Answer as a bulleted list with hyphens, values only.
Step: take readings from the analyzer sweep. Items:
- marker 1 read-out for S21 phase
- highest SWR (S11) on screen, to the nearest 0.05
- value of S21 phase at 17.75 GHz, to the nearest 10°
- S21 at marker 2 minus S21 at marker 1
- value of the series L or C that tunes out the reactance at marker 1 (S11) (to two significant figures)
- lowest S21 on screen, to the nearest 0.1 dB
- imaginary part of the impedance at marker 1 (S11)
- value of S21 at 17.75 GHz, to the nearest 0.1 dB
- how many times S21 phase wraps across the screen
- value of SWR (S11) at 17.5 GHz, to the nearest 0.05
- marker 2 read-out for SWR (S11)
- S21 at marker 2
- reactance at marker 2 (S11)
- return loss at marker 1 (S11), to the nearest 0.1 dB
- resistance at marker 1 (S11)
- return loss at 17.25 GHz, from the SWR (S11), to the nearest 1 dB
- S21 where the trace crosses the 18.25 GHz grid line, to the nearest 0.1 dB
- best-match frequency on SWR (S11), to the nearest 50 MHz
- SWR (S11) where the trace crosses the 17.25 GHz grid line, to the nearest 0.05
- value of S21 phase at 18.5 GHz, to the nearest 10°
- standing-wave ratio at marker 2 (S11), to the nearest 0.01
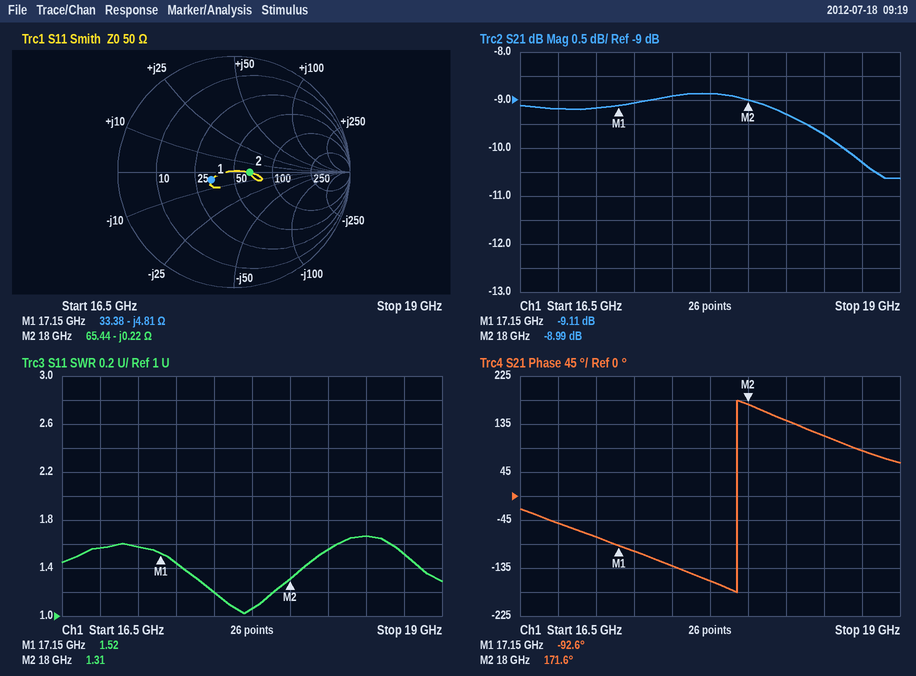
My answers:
- -92.6°
- 1.65
- -160°
- 0.12 dB
- 45 pH
- -10.6 dB
- -4.81 Ω
- -8.9 dB
- 1
- 1.20
- 1.31
- -8.99 dB
- -0.22 Ω
- 13.7 dB
- 33.38 Ω
- 15 dB
- -9.3 dB
- 17.70 GHz
- 1.45
- 110°
- 1.31
